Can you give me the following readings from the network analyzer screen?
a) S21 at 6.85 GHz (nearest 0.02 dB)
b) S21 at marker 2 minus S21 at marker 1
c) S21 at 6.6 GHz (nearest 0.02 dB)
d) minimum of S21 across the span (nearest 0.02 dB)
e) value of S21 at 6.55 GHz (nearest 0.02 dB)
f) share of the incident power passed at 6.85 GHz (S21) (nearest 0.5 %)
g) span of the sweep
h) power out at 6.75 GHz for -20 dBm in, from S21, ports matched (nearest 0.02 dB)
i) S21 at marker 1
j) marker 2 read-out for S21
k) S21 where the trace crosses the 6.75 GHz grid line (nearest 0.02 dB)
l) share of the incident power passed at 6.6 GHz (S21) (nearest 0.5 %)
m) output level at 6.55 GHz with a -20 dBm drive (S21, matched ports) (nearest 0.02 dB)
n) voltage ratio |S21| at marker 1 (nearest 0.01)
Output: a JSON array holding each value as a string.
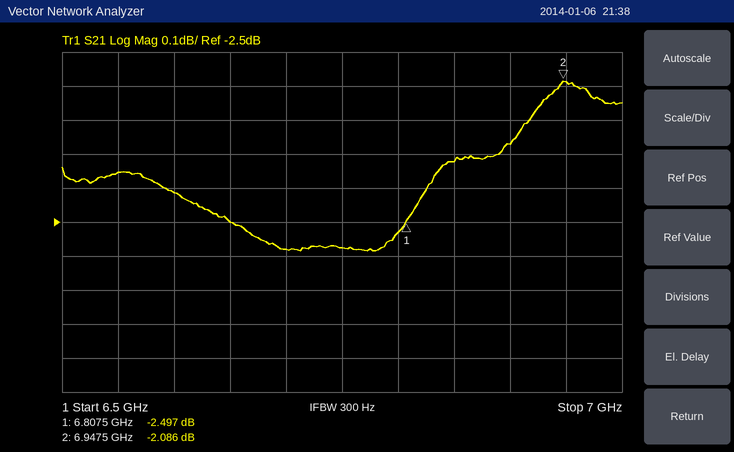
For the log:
["-2.32 dB", "0.411 dB", "-2.42 dB", "-2.58 dB", "-2.36 dB", "58.5 %", "500 MHz", "-22.58 dBm", "-2.497 dB", "-2.086 dB", "-2.58 dB", "57.5 %", "-22.36 dBm", "0.75"]
